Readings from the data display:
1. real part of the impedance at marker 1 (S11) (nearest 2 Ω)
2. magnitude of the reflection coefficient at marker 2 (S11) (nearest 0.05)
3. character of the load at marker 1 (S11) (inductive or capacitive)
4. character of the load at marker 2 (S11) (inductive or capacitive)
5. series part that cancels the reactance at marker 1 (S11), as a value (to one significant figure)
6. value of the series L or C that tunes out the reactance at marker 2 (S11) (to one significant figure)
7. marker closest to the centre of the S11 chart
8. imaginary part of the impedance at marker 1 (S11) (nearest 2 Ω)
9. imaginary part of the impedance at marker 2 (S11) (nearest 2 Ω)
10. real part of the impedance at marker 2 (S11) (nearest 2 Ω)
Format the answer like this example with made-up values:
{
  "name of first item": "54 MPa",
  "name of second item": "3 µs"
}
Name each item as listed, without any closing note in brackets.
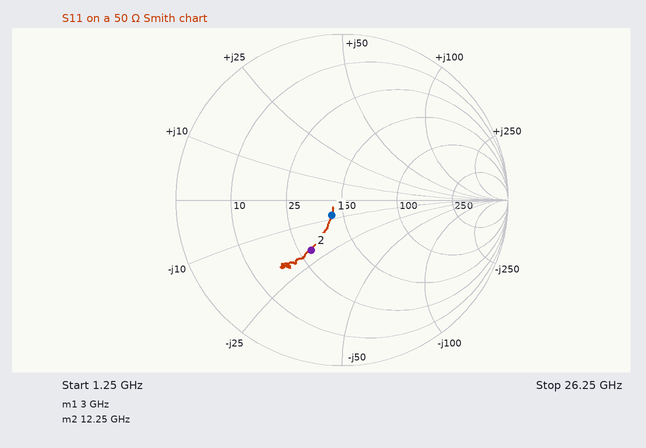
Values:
{
  "real part of the impedance at marker 1 (S11)": "44 Ω",
  "magnitude of the reflection coefficient at marker 2 (S11)": "0.35",
  "character of the load at marker 1 (S11)": "capacitive",
  "character of the load at marker 2 (S11)": "capacitive",
  "series part that cancels the reactance at marker 1 (S11), as a value": "400 pH",
  "value of the series L or C that tunes out the reactance at marker 2 (S11)": "300 pH",
  "marker closest to the centre of the S11 chart": "marker 1",
  "imaginary part of the impedance at marker 1 (S11)": "-8 Ω",
  "imaginary part of the impedance at marker 2 (S11)": "-20 Ω",
  "real part of the impedance at marker 2 (S11)": "30 Ω"
}
